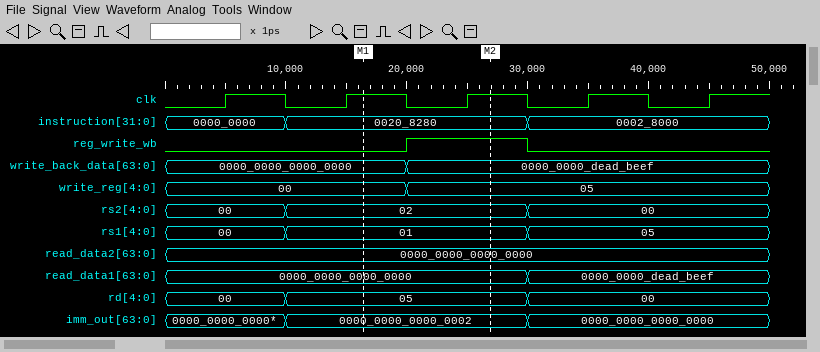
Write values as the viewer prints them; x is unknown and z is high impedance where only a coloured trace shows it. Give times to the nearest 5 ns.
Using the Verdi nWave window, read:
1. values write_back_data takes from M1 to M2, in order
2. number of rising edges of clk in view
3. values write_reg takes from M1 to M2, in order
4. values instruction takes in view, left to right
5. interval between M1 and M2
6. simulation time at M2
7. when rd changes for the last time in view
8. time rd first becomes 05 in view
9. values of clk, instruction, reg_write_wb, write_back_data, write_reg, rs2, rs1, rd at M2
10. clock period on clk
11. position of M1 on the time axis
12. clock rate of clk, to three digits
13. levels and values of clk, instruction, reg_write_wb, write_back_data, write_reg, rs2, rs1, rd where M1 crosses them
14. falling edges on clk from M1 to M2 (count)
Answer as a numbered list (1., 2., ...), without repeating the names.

1. 0000_0000_0000_0000, 0000_0000_dead_beef
2. 5
3. 00, 05
4. 0000_0000, 0020_8280, 0002_8000
5. 10 ns
6. 25 ns
7. 30 ns
8. 10 ns
9. clk=1, instruction=0020_8280, reg_write_wb=1, write_back_data=0000_0000_dead_beef, write_reg=05, rs2=02, rs1=01, rd=05
10. 10 ns
11. 15 ns
12. 100 MHz
13. clk=1, instruction=0020_8280, reg_write_wb=0, write_back_data=0000_0000_0000_0000, write_reg=00, rs2=02, rs1=01, rd=05
14. 1
